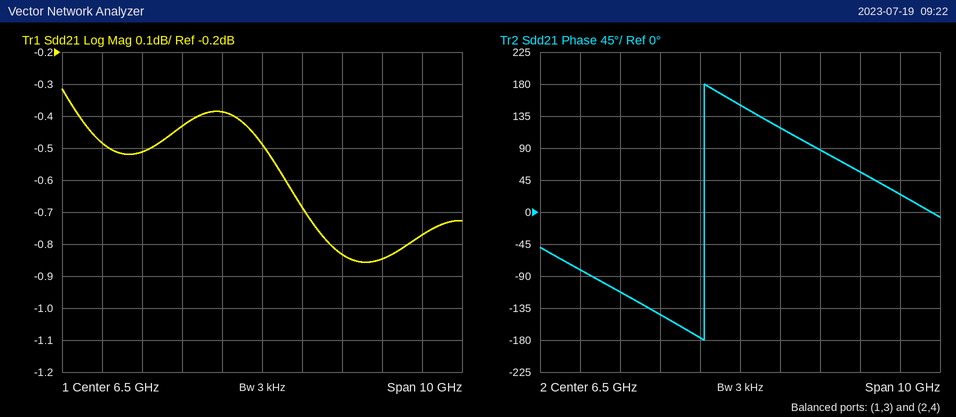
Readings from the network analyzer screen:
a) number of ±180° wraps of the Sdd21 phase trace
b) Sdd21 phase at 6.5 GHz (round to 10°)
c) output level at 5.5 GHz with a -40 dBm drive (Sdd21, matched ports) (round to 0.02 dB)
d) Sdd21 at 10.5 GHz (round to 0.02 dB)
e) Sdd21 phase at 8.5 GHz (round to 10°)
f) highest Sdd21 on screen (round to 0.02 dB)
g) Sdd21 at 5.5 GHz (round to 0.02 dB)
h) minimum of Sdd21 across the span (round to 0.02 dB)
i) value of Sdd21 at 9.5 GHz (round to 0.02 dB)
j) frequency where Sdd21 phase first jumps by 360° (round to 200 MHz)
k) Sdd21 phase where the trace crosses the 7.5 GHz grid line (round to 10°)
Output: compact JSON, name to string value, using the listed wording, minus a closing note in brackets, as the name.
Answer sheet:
{"number of ±180° wraps of the Sdd21 phase trace": "1", "Sdd21 phase at 6.5 GHz": "150°", "output level at 5.5 GHz with a -40 dBm drive (Sdd21, matched ports)": "-40.38 dBm", "Sdd21 at 10.5 GHz": "-0.78 dB", "Sdd21 phase at 8.5 GHz": "90°", "highest Sdd21 on screen": "-0.32 dB", "Sdd21 at 5.5 GHz": "-0.38 dB", "minimum of Sdd21 across the span": "-0.86 dB", "value of Sdd21 at 9.5 GHz": "-0.84 dB", "frequency where Sdd21 phase first jumps by 360°": "5.6 GHz", "Sdd21 phase where the trace crosses the 7.5 GHz grid line": "120°"}
